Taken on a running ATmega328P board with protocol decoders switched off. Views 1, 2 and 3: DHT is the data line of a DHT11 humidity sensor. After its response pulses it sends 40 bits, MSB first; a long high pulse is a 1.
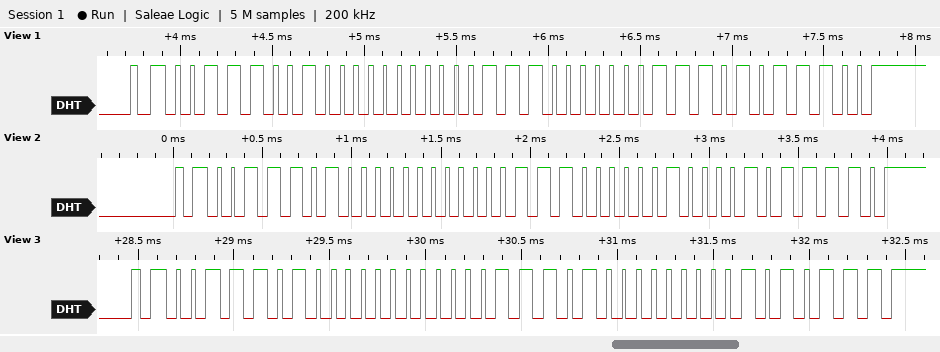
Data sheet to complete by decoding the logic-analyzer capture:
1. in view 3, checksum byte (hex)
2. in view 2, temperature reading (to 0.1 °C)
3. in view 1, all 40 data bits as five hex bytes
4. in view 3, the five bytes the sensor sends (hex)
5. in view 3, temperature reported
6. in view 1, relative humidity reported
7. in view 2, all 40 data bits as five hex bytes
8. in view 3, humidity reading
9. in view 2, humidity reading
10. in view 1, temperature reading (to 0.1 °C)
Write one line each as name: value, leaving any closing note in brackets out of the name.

in view 3, checksum byte: 0x57
in view 2, temperature reading: 28.8 °C
in view 1, all 40 data bits as five hex bytes: 39 00 1C 07 5C
in view 3, the five bytes the sensor sends: 3A 00 1D 00 57
in view 3, temperature reported: 29.0 °C
in view 1, relative humidity reported: 57 %
in view 2, all 40 data bits as five hex bytes: 3A 00 1C 08 5E
in view 3, humidity reading: 58 %
in view 2, humidity reading: 58 %
in view 1, temperature reading: 28.7 °C
